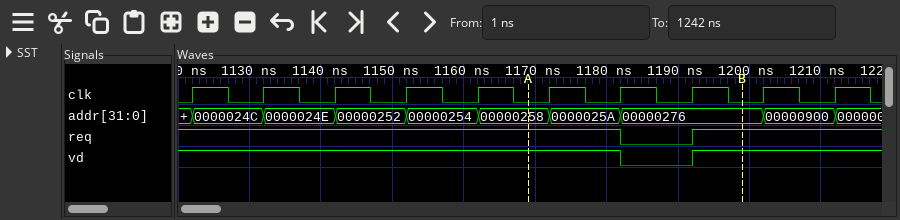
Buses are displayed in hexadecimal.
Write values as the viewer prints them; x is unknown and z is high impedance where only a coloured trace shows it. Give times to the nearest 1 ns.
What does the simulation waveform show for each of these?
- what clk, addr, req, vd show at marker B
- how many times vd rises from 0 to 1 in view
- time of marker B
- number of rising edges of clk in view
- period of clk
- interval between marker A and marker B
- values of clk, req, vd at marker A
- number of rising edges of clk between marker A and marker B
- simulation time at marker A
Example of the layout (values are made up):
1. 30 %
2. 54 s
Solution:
1. clk=0, addr=00000276, req=1, vd=1
2. 1
3. 1199 ns
4. 10
5. 10 ns
6. 30 ns
7. clk=0, req=1, vd=1
8. 3
9. 1169 ns
